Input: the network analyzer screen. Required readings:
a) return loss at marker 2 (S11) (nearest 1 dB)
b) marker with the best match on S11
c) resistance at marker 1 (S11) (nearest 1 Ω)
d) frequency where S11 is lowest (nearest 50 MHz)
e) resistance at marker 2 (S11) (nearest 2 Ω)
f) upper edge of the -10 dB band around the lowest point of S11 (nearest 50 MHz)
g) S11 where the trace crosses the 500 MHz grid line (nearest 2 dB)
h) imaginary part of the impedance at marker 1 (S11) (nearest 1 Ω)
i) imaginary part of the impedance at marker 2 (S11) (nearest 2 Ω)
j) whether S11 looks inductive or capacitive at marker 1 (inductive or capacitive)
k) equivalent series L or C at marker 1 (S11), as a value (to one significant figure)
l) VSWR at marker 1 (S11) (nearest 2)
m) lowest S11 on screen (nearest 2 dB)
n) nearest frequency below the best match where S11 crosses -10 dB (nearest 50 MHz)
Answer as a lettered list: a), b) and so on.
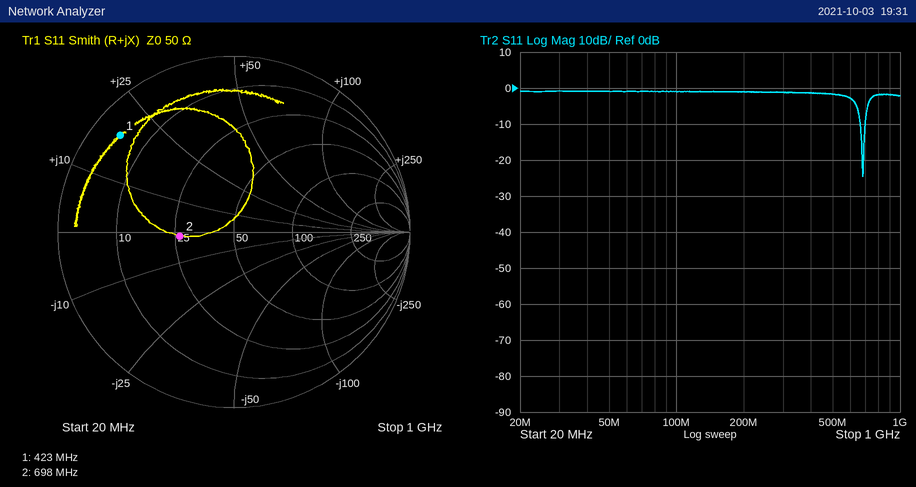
a) 10 dB
b) marker 2
c) 5 Ω
d) 700 MHz
e) 26 Ω
f) 700 MHz
g) -2 dB
h) +18 Ω
i) -2 Ω
j) inductive
k) 7 nH
l) 12
m) -24 dB
n) 650 MHz
